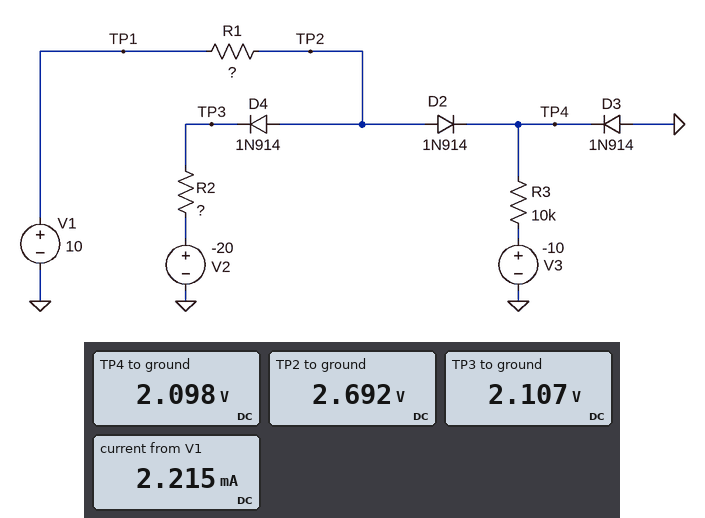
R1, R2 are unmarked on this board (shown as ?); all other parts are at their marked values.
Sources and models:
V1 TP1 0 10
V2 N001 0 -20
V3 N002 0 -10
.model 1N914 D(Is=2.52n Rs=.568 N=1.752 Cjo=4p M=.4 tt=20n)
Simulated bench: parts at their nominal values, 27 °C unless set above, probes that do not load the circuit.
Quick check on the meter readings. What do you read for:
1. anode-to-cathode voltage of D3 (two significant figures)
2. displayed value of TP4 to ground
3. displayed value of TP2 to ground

-2.1 V
2.098 V
2.692 V
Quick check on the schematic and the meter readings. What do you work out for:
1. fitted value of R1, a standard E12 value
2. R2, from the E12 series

3.3 kΩ
22 kΩ
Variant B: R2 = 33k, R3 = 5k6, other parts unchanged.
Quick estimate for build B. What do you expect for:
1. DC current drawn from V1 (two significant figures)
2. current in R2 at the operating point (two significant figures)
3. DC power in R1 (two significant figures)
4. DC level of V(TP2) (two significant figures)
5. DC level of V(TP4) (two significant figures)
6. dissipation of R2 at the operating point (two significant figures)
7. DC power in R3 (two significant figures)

2.6 mA
630 µA
22 mW
1.5 V
880 mV
13 mW
21 mW
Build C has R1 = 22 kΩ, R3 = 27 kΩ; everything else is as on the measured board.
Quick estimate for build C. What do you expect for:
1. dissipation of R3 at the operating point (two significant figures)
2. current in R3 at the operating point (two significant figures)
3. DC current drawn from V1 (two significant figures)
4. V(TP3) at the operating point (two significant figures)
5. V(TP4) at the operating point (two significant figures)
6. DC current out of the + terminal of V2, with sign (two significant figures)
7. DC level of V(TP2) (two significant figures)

3.3 mW
350 µA
670 µA
-5.3 V
-540 mV
-670 µA
-4.7 V
